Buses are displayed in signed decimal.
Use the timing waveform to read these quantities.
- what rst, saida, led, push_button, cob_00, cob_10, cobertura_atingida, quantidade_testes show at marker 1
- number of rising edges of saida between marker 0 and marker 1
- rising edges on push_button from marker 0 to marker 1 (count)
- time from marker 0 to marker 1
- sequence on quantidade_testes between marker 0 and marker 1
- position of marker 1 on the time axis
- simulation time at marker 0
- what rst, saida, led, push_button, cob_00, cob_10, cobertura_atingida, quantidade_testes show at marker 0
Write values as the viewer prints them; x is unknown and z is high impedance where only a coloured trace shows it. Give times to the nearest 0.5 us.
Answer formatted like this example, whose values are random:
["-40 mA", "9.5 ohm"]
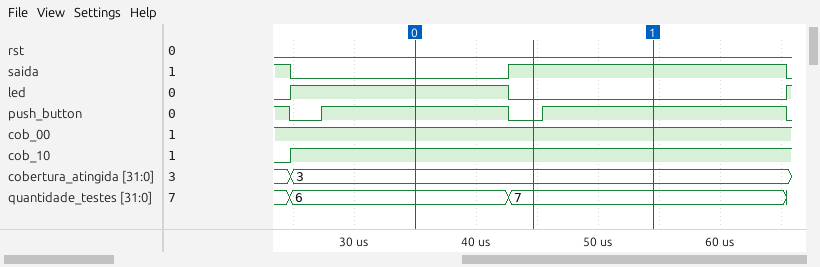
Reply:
["rst=0, saida=1, led=0, push_button=1, cob_00=1, cob_10=1, cobertura_atingida=3, quantidade_testes=7", "1", "1", "19.5 us", "6, 7", "54.5 us", "35 us", "rst=0, saida=0, led=1, push_button=1, cob_00=1, cob_10=1, cobertura_atingida=3, quantidade_testes=6"]
